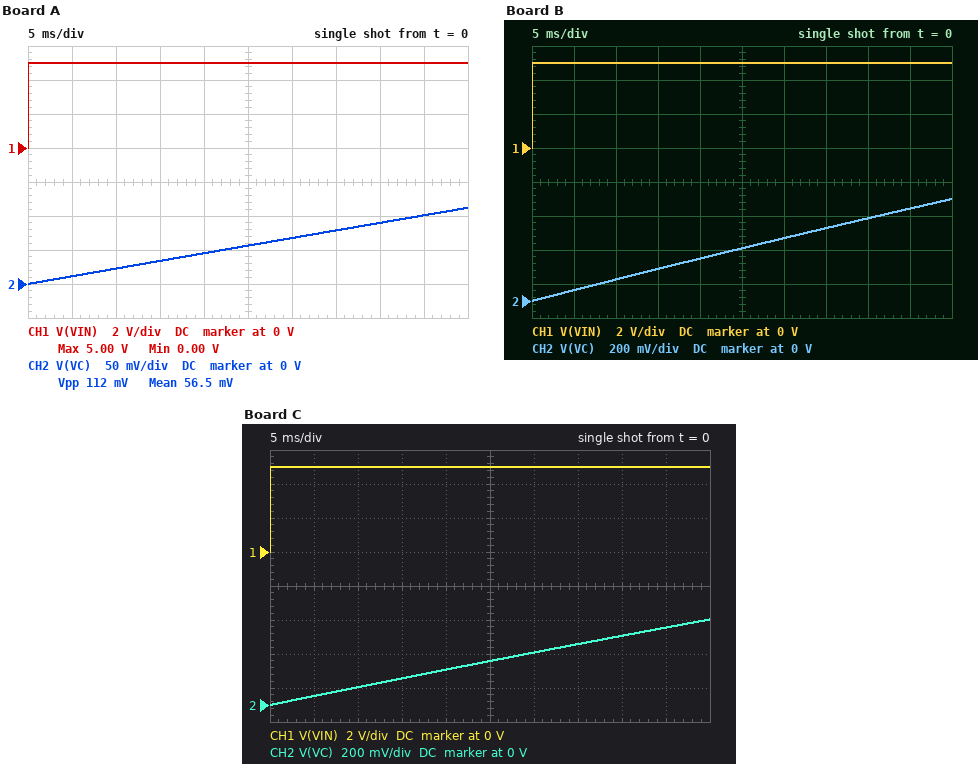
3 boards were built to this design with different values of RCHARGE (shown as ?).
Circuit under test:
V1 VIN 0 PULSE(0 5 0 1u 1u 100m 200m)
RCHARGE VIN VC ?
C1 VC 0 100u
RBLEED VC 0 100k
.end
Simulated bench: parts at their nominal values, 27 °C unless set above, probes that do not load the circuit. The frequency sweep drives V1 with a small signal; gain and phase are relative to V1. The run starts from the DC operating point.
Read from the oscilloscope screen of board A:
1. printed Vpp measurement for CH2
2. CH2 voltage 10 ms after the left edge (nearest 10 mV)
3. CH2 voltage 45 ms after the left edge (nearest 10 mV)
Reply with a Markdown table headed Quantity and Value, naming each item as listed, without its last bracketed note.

| Quantity | Value |
|---|---|
| printed Vpp measurement for CH2 | 112 mV |
| CH2 voltage 10 ms after the left edge | 20 mV |
| CH2 voltage 45 ms after the left edge | 100 mV |
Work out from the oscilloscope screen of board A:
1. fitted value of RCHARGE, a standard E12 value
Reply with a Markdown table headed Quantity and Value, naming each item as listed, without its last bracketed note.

| Quantity | Value |
|---|---|
| fitted value of RCHARGE, a standard E12 value | 22 kΩ |
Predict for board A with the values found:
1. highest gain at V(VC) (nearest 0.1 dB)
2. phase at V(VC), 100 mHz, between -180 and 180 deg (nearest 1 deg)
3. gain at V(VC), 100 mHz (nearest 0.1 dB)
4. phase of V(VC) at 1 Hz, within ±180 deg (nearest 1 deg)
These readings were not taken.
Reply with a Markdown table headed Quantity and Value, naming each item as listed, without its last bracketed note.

| Quantity | Value |
|---|---|
| highest gain at V(VC) | -1.7 dB |
| phase at V(VC), 100 mHz, between -180 and 180 deg | -49 deg |
| gain at V(VC), 100 mHz | -5.3 dB |
| phase of V(VC) at 1 Hz, within ±180 deg | -85 deg |
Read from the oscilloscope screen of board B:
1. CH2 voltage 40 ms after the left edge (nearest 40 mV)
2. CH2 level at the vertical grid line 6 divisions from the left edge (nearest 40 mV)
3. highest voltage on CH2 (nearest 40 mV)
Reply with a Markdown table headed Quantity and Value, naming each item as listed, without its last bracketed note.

| Quantity | Value |
|---|---|
| CH2 voltage 40 ms after the left edge | 480 mV |
| CH2 level at the vertical grid line 6 divisions from the left edge | 360 mV |
| highest voltage on CH2 | 600 mV |
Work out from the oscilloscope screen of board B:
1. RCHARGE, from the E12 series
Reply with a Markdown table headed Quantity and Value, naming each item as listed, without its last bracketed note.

| Quantity | Value |
|---|---|
| RCHARGE, from the E12 series | 3.9 kΩ |
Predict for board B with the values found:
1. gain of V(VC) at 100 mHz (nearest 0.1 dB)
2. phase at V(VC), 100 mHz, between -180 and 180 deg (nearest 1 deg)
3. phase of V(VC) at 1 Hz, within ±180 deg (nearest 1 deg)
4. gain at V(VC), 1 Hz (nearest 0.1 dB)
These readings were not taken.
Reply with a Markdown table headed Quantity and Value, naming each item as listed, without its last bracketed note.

| Quantity | Value |
|---|---|
| gain of V(VC) at 100 mHz | -0.6 dB |
| phase at V(VC), 100 mHz, between -180 and 180 deg | -13 deg |
| phase of V(VC) at 1 Hz, within ±180 deg | -67 deg |
| gain at V(VC), 1 Hz | -8.5 dB |
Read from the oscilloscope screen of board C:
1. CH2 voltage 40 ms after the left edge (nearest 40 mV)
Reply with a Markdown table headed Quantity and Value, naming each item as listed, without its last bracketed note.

| Quantity | Value |
|---|---|
| CH2 voltage 40 ms after the left edge | 400 mV |
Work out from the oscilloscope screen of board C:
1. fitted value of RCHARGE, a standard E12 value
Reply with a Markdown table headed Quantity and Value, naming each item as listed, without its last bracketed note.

| Quantity | Value |
|---|---|
| fitted value of RCHARGE, a standard E12 value | 4.7 kΩ |
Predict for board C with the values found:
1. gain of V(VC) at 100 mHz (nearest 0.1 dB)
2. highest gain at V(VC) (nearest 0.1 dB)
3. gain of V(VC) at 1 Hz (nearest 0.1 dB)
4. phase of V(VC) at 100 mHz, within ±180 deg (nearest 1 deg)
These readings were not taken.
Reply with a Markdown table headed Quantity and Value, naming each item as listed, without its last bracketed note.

| Quantity | Value |
|---|---|
| gain of V(VC) at 100 mHz | -0.7 dB |
| highest gain at V(VC) | -0.4 dB |
| gain of V(VC) at 1 Hz | -9.9 dB |
| phase of V(VC) at 100 mHz, within ±180 deg | -16 deg |
